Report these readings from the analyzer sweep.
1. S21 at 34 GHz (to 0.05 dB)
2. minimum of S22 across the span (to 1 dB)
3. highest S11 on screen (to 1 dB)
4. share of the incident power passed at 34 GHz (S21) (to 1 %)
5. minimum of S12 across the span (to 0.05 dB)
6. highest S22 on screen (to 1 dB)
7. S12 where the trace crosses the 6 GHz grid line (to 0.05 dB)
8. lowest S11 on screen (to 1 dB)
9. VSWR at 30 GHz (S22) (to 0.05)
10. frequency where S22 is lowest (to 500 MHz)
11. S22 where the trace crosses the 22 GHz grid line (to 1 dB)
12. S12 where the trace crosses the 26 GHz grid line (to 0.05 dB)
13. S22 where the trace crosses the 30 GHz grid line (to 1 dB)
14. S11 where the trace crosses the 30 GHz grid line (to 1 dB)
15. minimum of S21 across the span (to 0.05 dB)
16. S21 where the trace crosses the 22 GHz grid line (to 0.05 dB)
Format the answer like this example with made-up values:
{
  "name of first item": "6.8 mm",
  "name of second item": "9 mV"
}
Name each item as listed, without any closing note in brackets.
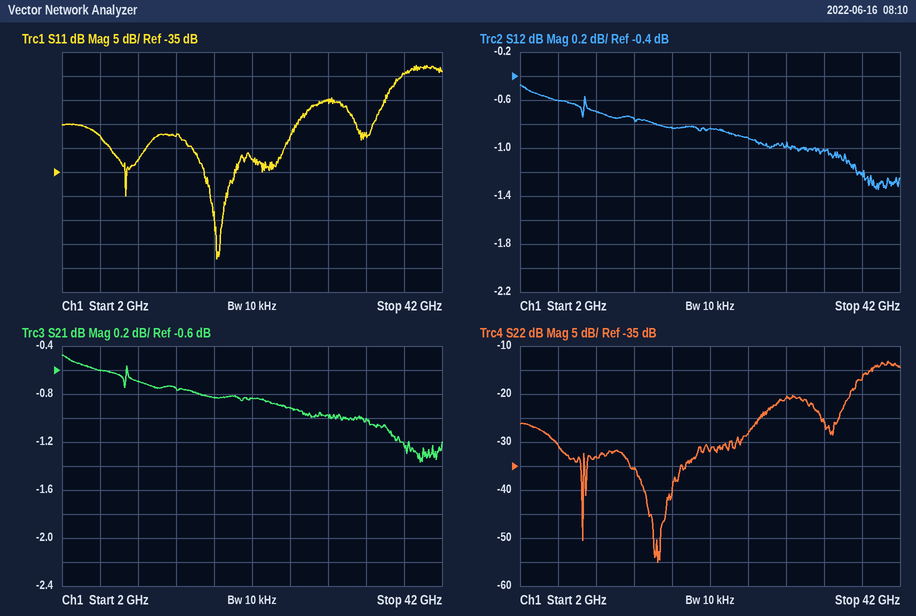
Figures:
{
  "S21 at 34 GHz": "-1.00 dB",
  "minimum of S22 across the span": "-55 dB",
  "highest S11 on screen": "-13 dB",
  "share of the incident power passed at 34 GHz (S21)": "79 %",
  "minimum of S12 across the span": "-1.35 dB",
  "highest S22 on screen": "-13 dB",
  "S12 where the trace crosses the 6 GHz grid line": "-0.60 dB",
  "lowest S11 on screen": "-53 dB",
  "VSWR at 30 GHz (S22)": "1.20",
  "frequency where S22 is lowest": "16.5 GHz",
  "S22 where the trace crosses the 22 GHz grid line": "-32 dB",
  "S12 where the trace crosses the 26 GHz grid line": "-0.90 dB",
  "S22 where the trace crosses the 30 GHz grid line": "-21 dB",
  "S11 where the trace crosses the 30 GHz grid line": "-20 dB",
  "minimum of S21 across the span": "-1.35 dB",
  "S21 where the trace crosses the 22 GHz grid line": "-0.85 dB"
}
